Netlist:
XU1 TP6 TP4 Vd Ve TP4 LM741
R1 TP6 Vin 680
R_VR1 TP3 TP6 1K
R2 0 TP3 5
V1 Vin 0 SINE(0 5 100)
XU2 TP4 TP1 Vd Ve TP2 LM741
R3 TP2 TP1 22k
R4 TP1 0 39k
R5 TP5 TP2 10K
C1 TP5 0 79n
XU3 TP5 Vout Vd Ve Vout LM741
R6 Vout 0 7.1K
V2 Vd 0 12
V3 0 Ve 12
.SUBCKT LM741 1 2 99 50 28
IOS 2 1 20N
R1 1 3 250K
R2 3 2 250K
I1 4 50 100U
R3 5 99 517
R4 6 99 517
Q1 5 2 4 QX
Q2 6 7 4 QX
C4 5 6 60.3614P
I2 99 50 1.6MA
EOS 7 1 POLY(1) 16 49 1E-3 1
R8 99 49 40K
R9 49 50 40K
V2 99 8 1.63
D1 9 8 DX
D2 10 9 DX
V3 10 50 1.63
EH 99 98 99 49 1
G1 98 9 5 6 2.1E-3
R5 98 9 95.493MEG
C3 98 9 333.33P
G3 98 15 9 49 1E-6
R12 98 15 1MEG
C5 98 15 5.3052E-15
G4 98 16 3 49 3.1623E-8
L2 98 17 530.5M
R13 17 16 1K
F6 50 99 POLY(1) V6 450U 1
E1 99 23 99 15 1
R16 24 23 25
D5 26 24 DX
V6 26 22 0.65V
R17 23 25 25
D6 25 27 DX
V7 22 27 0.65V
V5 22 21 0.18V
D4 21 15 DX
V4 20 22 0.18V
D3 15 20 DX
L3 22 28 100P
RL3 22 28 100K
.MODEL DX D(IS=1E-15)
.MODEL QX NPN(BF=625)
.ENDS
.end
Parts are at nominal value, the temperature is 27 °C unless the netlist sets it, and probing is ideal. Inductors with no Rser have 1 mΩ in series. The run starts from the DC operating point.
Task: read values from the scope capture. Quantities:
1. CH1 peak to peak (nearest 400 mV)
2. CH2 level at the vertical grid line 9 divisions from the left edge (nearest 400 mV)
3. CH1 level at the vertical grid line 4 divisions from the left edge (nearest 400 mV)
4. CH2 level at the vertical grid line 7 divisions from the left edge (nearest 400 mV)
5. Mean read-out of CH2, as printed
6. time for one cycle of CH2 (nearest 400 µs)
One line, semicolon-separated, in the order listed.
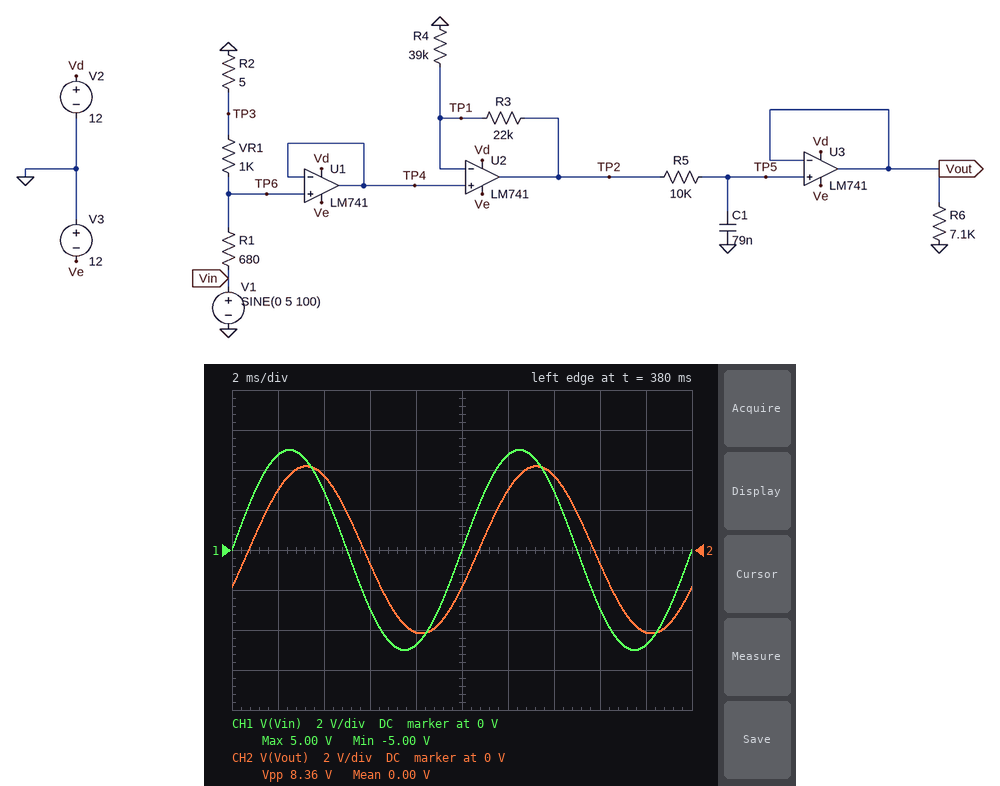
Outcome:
10.0 V; -4.0 V; -4.8 V; 3.6 V; 0.00 V; 10.0 ms
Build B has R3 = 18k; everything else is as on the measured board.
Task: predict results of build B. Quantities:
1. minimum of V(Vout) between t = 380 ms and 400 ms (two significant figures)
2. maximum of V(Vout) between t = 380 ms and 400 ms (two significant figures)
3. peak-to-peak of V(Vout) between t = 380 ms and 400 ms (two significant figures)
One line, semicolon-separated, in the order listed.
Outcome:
-3.9 V; 3.9 V; 7.8 V
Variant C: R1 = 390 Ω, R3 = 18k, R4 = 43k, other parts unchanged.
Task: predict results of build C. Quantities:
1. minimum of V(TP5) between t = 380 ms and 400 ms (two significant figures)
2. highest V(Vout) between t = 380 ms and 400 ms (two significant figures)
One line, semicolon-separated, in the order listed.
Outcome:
-4.6 V; 4.6 V
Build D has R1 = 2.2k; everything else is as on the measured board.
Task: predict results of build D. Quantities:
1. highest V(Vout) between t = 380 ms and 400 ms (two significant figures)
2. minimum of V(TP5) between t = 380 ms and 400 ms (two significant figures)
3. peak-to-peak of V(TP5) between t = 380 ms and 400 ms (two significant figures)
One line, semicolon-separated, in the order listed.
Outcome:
2.2 V; -2.2 V; 4.4 V
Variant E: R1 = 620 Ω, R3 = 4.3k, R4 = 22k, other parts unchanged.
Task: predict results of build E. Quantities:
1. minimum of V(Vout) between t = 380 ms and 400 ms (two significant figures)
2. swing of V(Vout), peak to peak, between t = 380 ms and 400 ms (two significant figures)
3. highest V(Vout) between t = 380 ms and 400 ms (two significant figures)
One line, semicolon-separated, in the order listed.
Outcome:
-3.3 V; 6.6 V; 3.3 V
